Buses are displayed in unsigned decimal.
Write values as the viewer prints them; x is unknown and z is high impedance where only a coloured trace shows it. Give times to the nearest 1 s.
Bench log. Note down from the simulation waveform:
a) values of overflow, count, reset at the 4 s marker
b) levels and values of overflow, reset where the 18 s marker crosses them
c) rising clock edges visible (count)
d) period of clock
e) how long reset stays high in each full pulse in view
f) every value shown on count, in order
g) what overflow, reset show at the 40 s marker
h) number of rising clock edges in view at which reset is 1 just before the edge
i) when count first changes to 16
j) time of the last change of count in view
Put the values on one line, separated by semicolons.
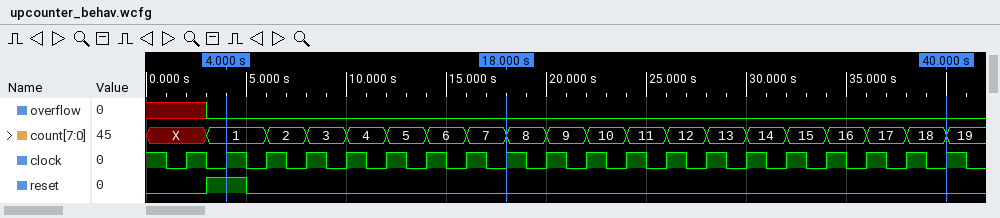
overflow=0, count=1, reset=1; overflow=0, reset=0; 20; 2 s; 2 s; X, 1, 2, 3, 4, 5, 6, 7, 8, 9, 10, 11, 12, 13, 14, 15, 16, 17, 18, 19; overflow=0, reset=0; 1; 34 s; 40 s
